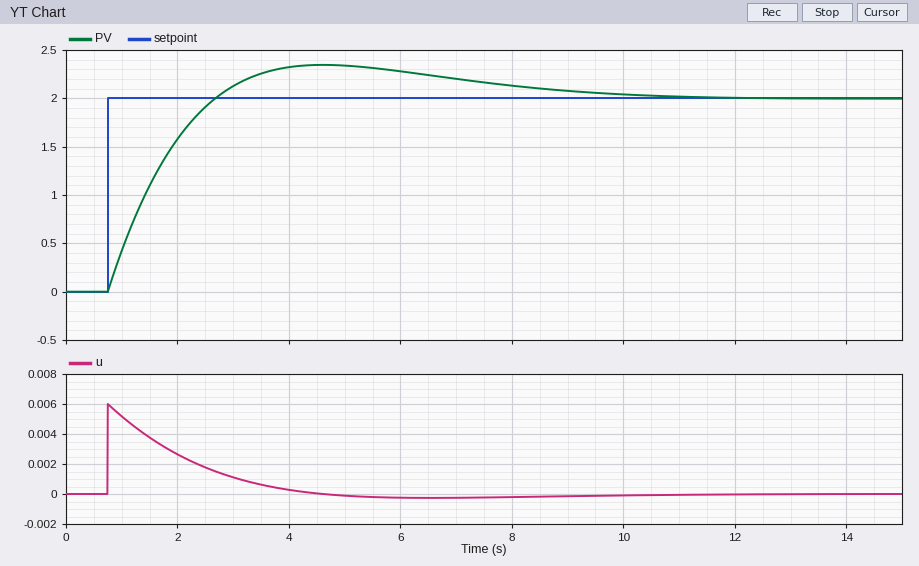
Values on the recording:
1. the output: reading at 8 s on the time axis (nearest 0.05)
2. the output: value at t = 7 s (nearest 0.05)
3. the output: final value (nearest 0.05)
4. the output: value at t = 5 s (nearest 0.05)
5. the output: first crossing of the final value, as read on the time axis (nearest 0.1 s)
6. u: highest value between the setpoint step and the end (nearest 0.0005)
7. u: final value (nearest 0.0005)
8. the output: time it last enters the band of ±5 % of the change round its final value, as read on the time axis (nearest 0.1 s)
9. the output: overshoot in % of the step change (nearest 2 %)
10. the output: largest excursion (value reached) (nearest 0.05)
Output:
2.15
2.20
2.00
2.35
2.7 s
0.0060
0.0000
8.5 s
18 %
2.35
